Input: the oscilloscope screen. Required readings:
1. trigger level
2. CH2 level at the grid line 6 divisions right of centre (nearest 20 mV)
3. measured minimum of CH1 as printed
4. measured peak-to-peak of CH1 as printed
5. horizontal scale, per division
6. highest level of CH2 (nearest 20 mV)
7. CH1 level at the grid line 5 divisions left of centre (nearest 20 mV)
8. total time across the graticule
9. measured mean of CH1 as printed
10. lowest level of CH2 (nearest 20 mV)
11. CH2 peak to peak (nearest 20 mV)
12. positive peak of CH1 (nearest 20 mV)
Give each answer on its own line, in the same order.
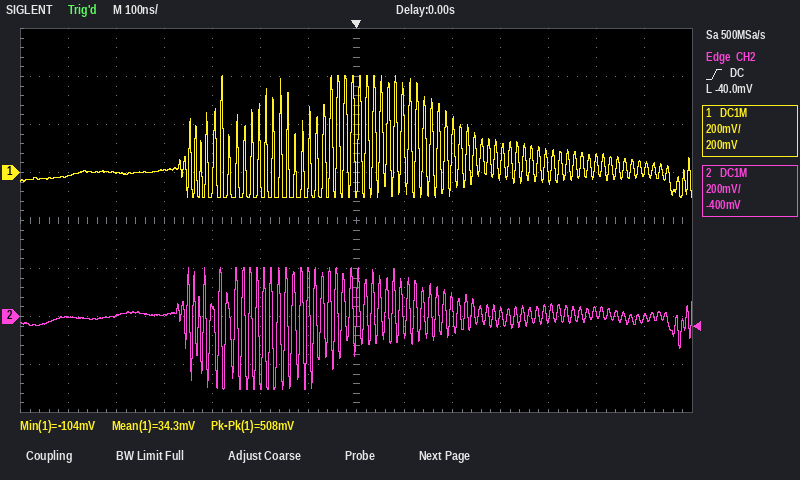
-40.0 mV
0 mV
-104 mV
508 mV
100 ns
200 mV
0 mV
1.4 µs
34.3 mV
-300 mV
500 mV
400 mV
